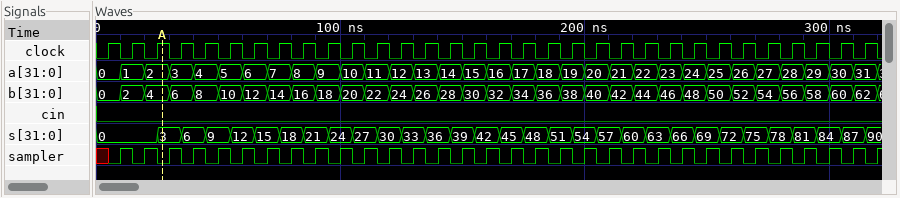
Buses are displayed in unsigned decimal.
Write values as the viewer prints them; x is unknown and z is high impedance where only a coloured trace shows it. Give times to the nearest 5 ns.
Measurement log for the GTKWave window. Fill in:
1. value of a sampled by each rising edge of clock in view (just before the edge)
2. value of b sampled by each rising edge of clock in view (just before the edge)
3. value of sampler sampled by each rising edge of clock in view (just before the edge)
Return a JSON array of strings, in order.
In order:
["0, 1, 2, 3, 4, 5, 6, 7, 8, 9, 10, 11, 12, 13, 14, 15, 16, 17, 18, 19, 20, 21, 22, 23, 24, 25, 26, 27, 28, 29, 30, 31", "0, 2, 4, 6, 8, 10, 12, 14, 16, 18, 20, 22, 24, 26, 28, 30, 32, 34, 36, 38, 40, 42, 44, 46, 48, 50, 52, 54, 56, 58, 60, 62", "x 1 1 1 1 1 1 1 1 1 1 1 1 1 1 1 1 1 1 1 1 1 1 1 1 1 1 1 1 1 1 1"]
